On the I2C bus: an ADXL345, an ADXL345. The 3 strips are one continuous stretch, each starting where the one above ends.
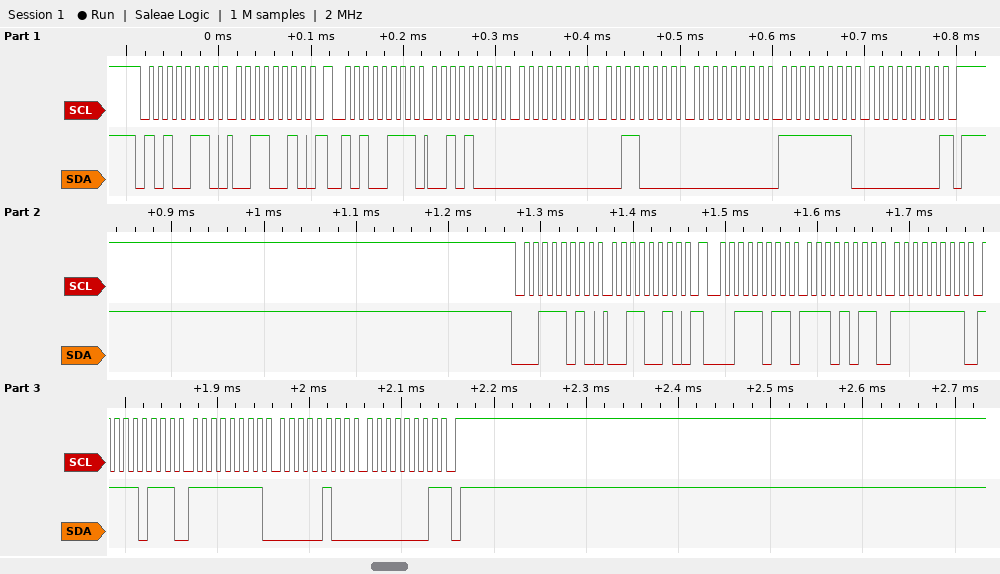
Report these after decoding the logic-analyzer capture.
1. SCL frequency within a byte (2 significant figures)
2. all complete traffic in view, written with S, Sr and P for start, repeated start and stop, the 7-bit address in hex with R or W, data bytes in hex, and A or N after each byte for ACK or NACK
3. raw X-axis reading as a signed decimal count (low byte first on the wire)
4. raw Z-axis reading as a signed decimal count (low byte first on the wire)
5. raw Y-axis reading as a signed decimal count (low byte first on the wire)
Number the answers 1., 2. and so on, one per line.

1. 100 kHz
2. S 53W A 32 A Sr 53R A 28 A 00 A 30 A 00 A FF A 00 N P S 1DW A 32 A Sr 1DR A EB A FF A F7 A FF A 04 A 01 N P
3. 40
4. 255
5. 48
